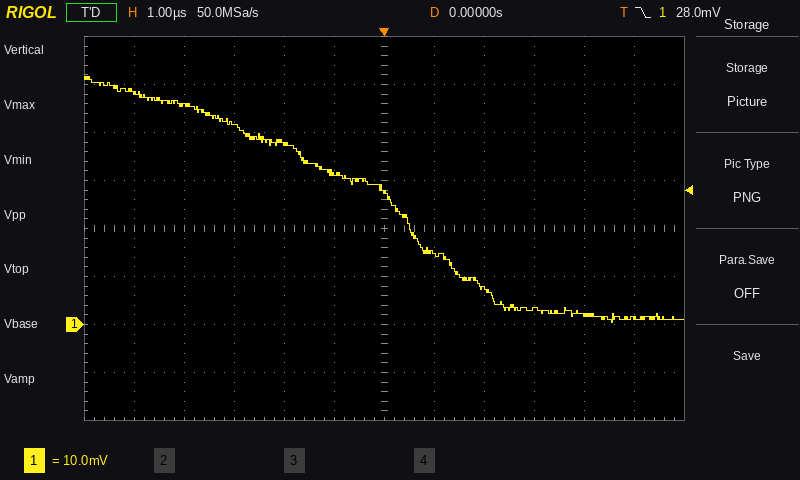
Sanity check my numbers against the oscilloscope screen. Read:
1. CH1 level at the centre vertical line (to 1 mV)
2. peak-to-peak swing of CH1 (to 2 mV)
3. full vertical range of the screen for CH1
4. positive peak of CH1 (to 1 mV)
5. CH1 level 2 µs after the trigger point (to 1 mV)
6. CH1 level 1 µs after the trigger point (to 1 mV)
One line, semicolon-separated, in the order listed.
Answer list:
28 mV; 52 mV; 80 mV; 52 mV; 7 mV; 15 mV
